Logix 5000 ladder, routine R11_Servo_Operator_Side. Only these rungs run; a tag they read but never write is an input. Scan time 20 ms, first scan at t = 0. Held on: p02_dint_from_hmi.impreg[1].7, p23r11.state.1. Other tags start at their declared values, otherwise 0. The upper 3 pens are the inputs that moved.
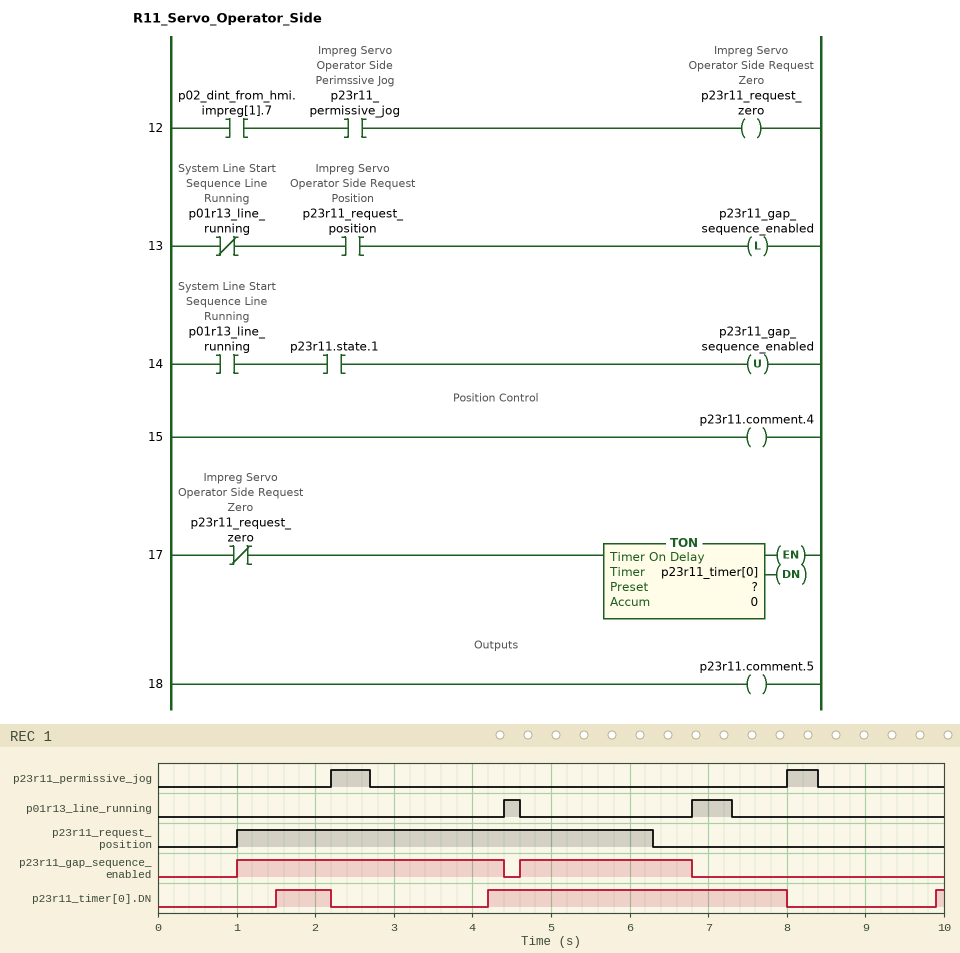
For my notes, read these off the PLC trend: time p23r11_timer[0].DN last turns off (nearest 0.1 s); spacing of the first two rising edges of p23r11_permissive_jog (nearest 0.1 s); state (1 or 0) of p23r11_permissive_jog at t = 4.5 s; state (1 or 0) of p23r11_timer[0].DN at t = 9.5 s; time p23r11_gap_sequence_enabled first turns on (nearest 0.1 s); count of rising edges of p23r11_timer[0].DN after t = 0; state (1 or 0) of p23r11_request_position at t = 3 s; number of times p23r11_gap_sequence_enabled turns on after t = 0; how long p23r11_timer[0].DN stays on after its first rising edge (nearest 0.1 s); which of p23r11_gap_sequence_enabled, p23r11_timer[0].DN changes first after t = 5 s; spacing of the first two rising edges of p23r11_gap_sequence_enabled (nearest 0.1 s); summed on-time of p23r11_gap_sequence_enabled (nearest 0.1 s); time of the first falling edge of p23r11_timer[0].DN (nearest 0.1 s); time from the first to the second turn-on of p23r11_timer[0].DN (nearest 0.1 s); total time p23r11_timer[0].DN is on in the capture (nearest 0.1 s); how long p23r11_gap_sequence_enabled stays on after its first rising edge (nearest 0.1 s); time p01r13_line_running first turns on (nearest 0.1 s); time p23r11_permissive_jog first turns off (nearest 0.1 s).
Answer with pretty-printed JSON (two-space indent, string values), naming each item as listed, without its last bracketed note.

{
  "time p23r11_timer[0].DN last turns off": "8.0 s",
  "spacing of the first two rising edges of p23r11_permissive_jog": "5.8 s",
  "state (1 or 0) of p23r11_permissive_jog at t = 4.5 s": "0",
  "state (1 or 0) of p23r11_timer[0].DN at t = 9.5 s": "0",
  "time p23r11_gap_sequence_enabled first turns on": "1.0 s",
  "count of rising edges of p23r11_timer[0].DN after t = 0": "3",
  "state (1 or 0) of p23r11_request_position at t = 3 s": "1",
  "number of times p23r11_gap_sequence_enabled turns on after t = 0": "2",
  "how long p23r11_timer[0].DN stays on after its first rising edge": "0.7 s",
  "which of p23r11_gap_sequence_enabled, p23r11_timer[0].DN changes first after t = 5 s": "p23r11_gap_sequence_enabled",
  "spacing of the first two rising edges of p23r11_gap_sequence_enabled": "3.6 s",
  "summed on-time of p23r11_gap_sequence_enabled": "5.6 s",
  "time of the first falling edge of p23r11_timer[0].DN": "2.2 s",
  "time from the first to the second turn-on of p23r11_timer[0].DN": "2.7 s",
  "total time p23r11_timer[0].DN is on in the capture": "4.6 s",
  "how long p23r11_gap_sequence_enabled stays on after its first rising edge": "3.4 s",
  "time p01r13_line_running first turns on": "4.4 s",
  "time p23r11_permissive_jog first turns off": "2.7 s"
}
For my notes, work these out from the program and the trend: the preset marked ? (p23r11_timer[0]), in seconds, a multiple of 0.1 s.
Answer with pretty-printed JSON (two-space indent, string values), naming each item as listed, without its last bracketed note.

{
  "the preset marked ? (p23r11_timer[0]), in seconds, a multiple of 0.1 s": "1.5 s"
}
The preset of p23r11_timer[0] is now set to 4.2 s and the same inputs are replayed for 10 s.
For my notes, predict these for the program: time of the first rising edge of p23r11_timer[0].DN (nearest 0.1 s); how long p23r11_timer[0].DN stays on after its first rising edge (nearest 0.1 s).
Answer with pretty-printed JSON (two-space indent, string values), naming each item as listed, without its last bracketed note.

{
  "time of the first rising edge of p23r11_timer[0].DN": "6.9 s",
  "how long p23r11_timer[0].DN stays on after its first rising edge": "1.1 s"
}
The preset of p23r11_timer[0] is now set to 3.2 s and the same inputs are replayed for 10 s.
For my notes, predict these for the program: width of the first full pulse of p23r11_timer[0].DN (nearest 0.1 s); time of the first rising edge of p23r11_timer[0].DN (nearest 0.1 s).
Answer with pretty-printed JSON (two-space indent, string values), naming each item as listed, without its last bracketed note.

{
  "width of the first full pulse of p23r11_timer[0].DN": "2.1 s",
  "time of the first rising edge of p23r11_timer[0].DN": "5.9 s"
}
